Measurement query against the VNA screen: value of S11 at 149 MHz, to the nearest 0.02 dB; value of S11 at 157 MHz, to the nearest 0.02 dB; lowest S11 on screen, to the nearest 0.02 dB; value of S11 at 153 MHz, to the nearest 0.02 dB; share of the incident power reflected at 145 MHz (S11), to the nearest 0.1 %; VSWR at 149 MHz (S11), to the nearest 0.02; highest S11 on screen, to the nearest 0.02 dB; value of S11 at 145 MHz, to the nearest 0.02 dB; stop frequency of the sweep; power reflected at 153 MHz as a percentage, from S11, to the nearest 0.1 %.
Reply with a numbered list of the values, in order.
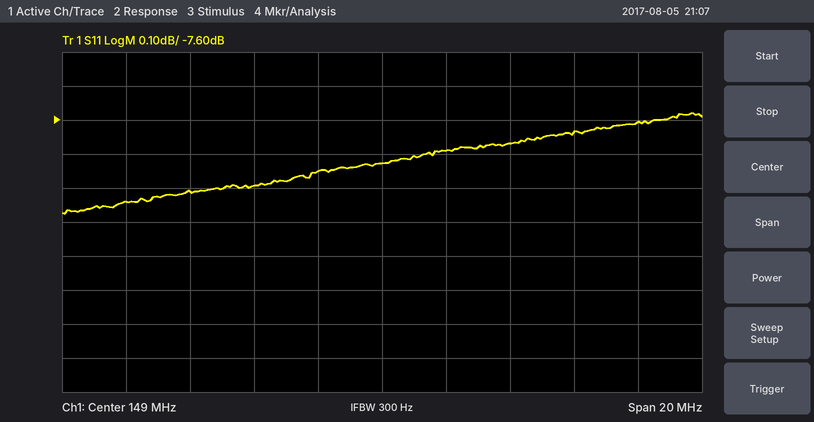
1. -7.72 dB
2. -7.60 dB
3. -7.88 dB
4. -7.66 dB
5. 16.6 %
6. 2.40
7. -7.58 dB
8. -7.80 dB
9. 159 MHz
10. 17.1 %
